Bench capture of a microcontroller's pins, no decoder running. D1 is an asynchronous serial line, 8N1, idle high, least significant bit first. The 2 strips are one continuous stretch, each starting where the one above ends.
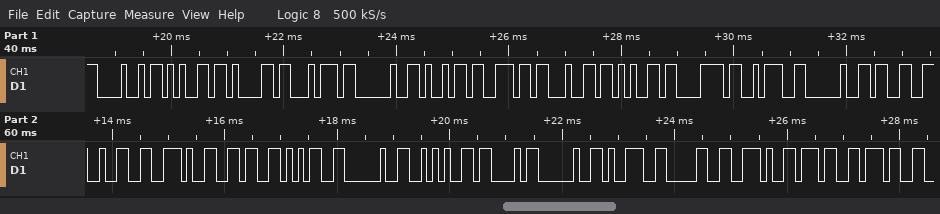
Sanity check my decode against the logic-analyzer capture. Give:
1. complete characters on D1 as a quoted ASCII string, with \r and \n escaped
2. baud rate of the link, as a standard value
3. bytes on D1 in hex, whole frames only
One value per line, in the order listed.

"Heat index: 32.65 *C 90.77"
9600 baud
48 65 61 74 20 69 6E 64 65 78 3A 20 33 32 2E 36 35 20 2A 43 20 39 30 2E 37 37
